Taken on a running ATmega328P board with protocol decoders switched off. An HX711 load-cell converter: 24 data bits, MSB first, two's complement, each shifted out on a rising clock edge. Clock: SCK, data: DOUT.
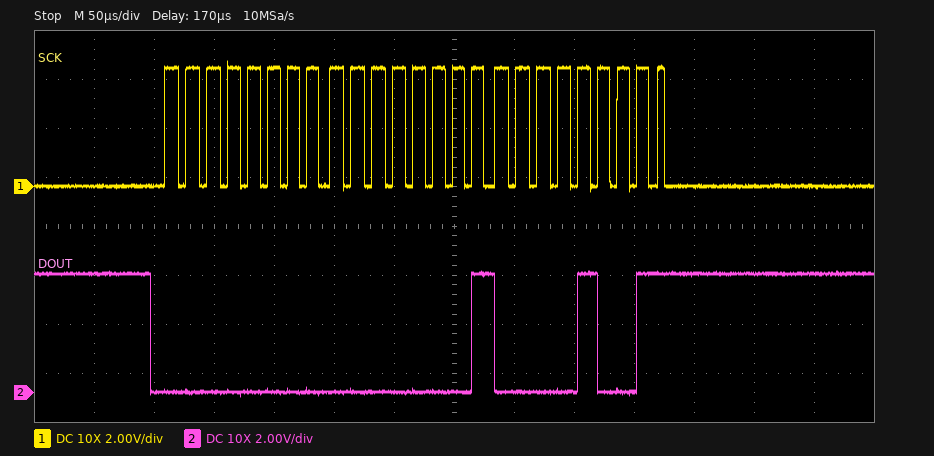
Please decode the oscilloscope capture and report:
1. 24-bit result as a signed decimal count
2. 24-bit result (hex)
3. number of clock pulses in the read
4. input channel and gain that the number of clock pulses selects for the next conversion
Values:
265
0x000109
25
channel A, gain 128
